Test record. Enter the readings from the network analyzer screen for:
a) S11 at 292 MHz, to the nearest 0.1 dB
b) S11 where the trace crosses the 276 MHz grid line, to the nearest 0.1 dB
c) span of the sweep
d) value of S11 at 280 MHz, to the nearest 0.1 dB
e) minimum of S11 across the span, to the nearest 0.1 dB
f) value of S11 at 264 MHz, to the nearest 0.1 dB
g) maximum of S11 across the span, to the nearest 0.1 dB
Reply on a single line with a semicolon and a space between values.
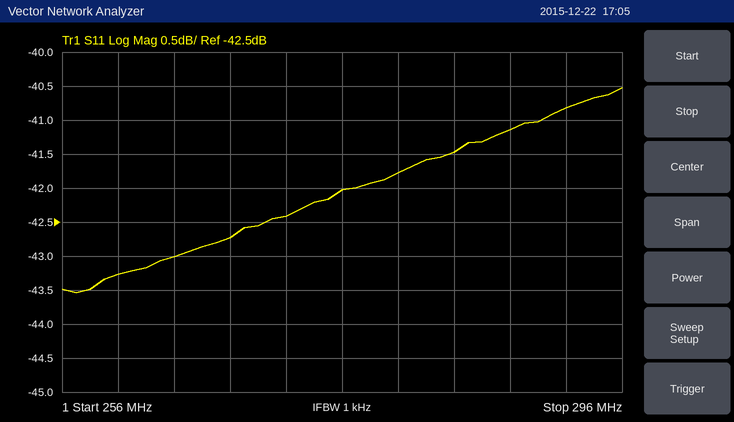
-40.8 dB; -42.0 dB; 40 MHz; -41.8 dB; -43.5 dB; -43.0 dB; -40.5 dB
